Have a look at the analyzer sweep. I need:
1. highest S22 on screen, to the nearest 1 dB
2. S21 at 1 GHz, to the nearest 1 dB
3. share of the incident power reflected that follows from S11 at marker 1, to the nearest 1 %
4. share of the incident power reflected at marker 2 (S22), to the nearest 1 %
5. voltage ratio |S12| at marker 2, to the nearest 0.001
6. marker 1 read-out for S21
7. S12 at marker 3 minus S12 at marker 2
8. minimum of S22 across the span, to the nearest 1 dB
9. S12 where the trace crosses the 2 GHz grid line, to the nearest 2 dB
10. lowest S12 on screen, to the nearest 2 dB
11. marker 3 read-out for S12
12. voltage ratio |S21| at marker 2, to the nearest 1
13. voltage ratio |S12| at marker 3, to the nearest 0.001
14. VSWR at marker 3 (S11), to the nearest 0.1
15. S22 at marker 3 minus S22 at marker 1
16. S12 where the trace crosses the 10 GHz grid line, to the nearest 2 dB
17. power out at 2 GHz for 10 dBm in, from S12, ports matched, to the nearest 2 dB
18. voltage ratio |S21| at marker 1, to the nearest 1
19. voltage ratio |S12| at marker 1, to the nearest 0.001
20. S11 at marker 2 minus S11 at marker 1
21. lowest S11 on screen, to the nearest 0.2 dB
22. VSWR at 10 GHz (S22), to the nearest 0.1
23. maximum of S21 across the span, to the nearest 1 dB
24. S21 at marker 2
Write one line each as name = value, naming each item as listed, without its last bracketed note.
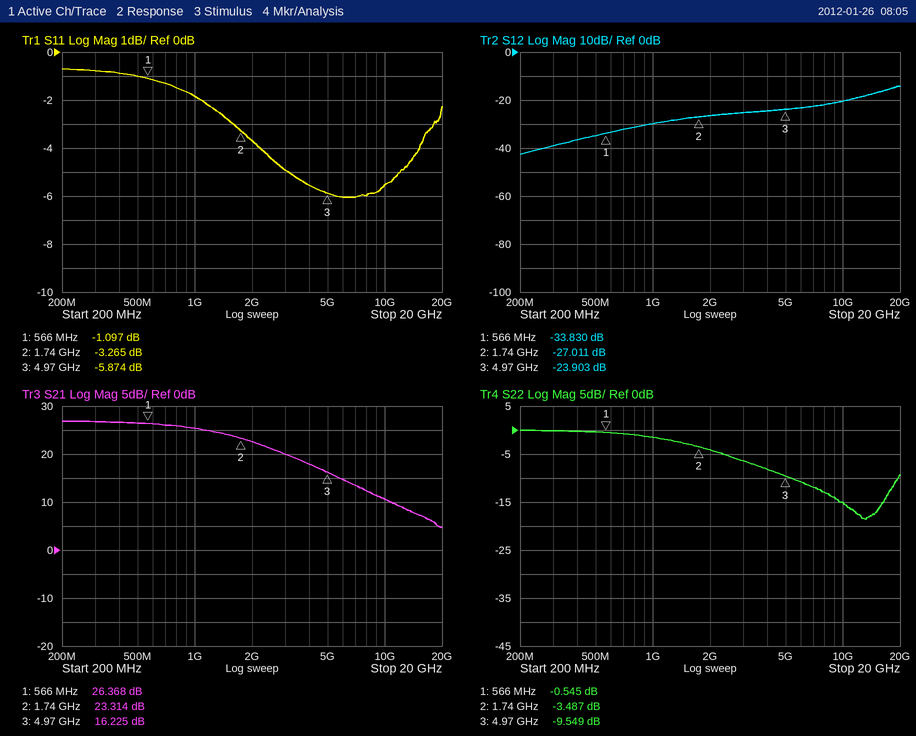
highest S22 on screen, to the nearest 1 dB = 0 dB
S21 at 1 GHz, to the nearest 1 dB = 25 dB
share of the incident power reflected that follows from S11 at marker 1, to the nearest 1 % = 78 %
share of the incident power reflected at marker 2 (S22), to the nearest 1 % = 45 %
voltage ratio |S12| at marker 2, to the nearest 0.001 = 0.045
marker 1 read-out for S21 = 26.368 dB
S12 at marker 3 minus S12 at marker 2 = 3.108 dB
minimum of S22 across the span, to the nearest 1 dB = -19 dB
S12 where the trace crosses the 2 GHz grid line, to the nearest 2 dB = -26 dB
lowest S12 on screen, to the nearest 2 dB = -42 dB
marker 3 read-out for S12 = -23.903 dB
voltage ratio |S21| at marker 2, to the nearest 1 = 15
voltage ratio |S12| at marker 3, to the nearest 0.001 = 0.064
VSWR at marker 3 (S11), to the nearest 0.1 = 3.1
S22 at marker 3 minus S22 at marker 1 = -9.004 dB
S12 where the trace crosses the 10 GHz grid line, to the nearest 2 dB = -20 dB
power out at 2 GHz for 10 dBm in, from S12, ports matched, to the nearest 2 dB = -16 dBm
voltage ratio |S21| at marker 1, to the nearest 1 = 21
voltage ratio |S12| at marker 1, to the nearest 0.001 = 0.020
S11 at marker 2 minus S11 at marker 1 = -2.168 dB
lowest S11 on screen, to the nearest 0.2 dB = -6.0 dB
VSWR at 10 GHz (S22), to the nearest 0.1 = 1.4
maximum of S21 across the span, to the nearest 1 dB = 27 dB
S21 at marker 2 = 23.314 dB
